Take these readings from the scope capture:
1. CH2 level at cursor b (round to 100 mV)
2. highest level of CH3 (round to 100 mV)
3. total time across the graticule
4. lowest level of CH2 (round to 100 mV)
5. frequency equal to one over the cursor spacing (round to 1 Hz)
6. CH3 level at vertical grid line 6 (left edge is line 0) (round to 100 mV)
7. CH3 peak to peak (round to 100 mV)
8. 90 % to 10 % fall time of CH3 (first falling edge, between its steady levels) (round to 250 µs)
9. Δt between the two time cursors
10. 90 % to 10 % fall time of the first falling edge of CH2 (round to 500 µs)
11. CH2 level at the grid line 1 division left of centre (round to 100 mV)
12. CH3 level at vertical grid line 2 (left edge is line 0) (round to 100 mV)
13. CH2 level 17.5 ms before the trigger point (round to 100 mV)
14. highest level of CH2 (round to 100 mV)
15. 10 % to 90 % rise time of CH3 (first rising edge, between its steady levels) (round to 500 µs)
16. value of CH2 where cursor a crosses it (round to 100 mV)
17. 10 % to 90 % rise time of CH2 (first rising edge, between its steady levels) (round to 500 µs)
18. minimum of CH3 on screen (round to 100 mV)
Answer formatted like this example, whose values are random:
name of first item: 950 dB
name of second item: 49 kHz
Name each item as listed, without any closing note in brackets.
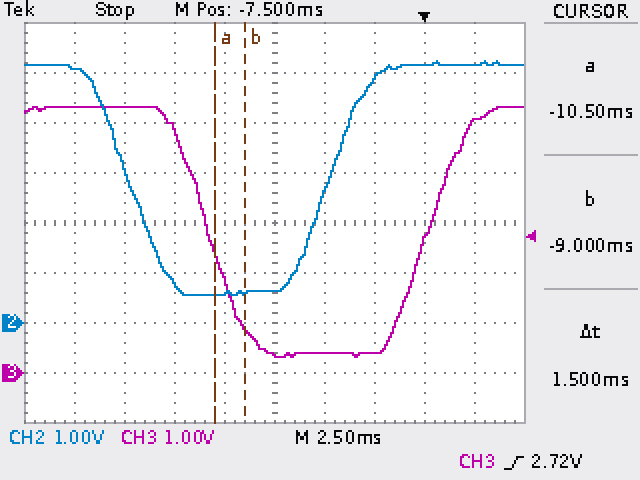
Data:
CH2 level at cursor b: 600 mV
highest level of CH3: 5.3 V
total time across the graticule: 25 ms
lowest level of CH2: 600 mV
frequency equal to one over the cursor spacing: 667 Hz
CH3 level at vertical grid line 6 (left edge is line 0): 400 mV
CH3 peak to peak: 5.0 V
90 % to 10 % fall time of CH3 (first falling edge, between its steady levels): 3.50 ms
Δt between the two time cursors: 1.5 ms
90 % to 10 % fall time of the first falling edge of CH2: 3.5 ms
CH2 level at the grid line 1 division left of centre: 600 mV
CH3 level at vertical grid line 2 (left edge is line 0): 5.3 V
CH2 level 17.5 ms before the trigger point: 5.1 V
highest level of CH2: 5.2 V
10 % to 90 % rise time of CH3 (first rising edge, between its steady levels): 3.5 ms
value of CH2 where cursor a crosses it: 600 mV
10 % to 90 % rise time of CH2 (first rising edge, between its steady levels): 3.5 ms
minimum of CH3 on screen: 300 mV
